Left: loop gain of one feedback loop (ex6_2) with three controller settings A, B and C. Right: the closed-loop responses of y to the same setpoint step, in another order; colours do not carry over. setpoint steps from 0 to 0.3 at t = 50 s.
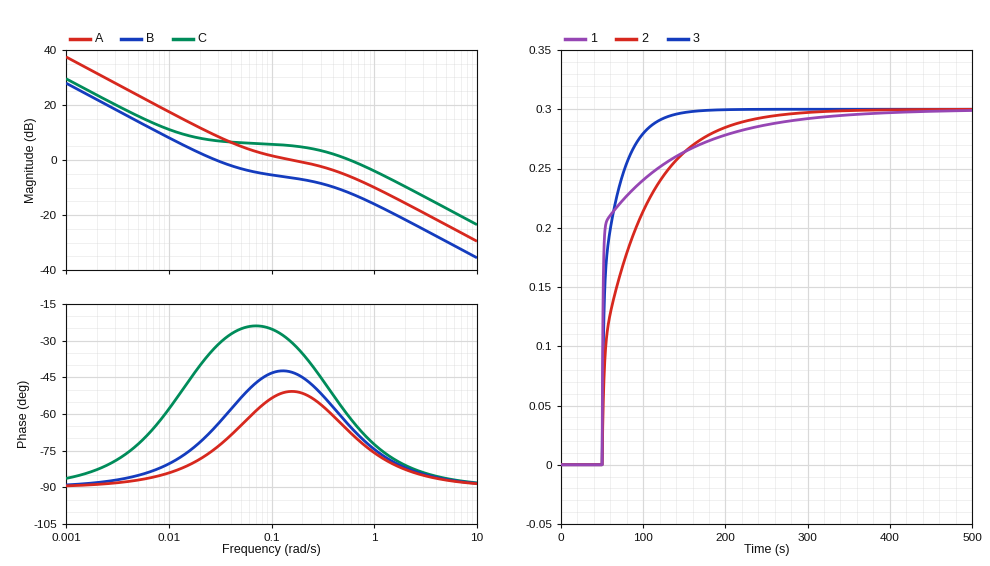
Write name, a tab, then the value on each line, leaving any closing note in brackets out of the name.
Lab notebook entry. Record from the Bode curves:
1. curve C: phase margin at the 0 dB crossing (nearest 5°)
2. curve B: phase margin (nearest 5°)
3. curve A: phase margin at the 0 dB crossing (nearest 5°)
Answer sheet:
curve C: phase margin at the 0 dB crossing	120°
curve B: phase margin	115°
curve A: phase margin at the 0 dB crossing	130°
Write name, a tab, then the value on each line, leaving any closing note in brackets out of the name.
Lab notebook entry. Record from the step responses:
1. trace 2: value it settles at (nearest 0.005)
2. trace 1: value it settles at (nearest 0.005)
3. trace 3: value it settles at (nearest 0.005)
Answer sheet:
trace 2: value it settles at	0.300
trace 1: value it settles at	0.300
trace 3: value it settles at	0.300
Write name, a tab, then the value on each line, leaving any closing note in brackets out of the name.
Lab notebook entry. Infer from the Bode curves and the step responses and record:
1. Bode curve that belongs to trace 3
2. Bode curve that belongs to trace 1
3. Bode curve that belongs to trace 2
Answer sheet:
Bode curve that belongs to trace 3	A
Bode curve that belongs to trace 1	C
Bode curve that belongs to trace 2	B
